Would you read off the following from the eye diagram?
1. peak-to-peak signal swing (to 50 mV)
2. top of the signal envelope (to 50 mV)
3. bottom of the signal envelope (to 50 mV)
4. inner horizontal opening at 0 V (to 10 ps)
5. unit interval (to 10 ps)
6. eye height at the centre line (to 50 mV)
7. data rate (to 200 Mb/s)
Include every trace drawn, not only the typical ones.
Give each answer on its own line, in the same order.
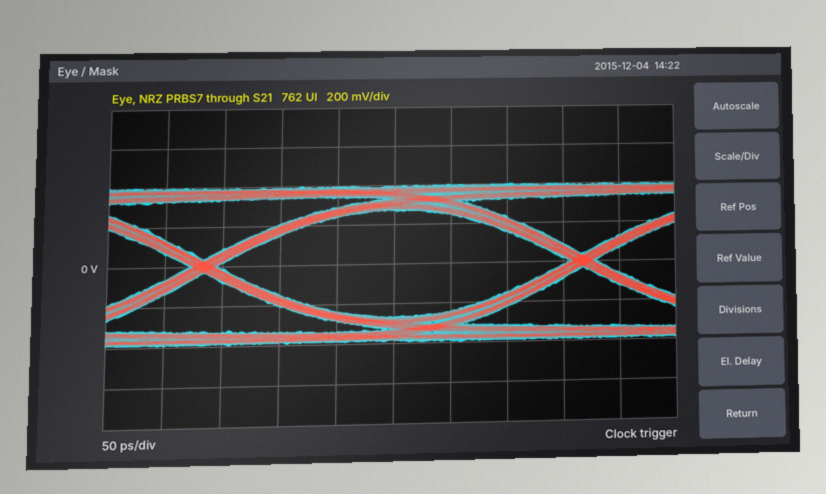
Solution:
800 mV
400 mV
-400 mV
310 ps
330 ps
550 mV
3.0 Gb/s
